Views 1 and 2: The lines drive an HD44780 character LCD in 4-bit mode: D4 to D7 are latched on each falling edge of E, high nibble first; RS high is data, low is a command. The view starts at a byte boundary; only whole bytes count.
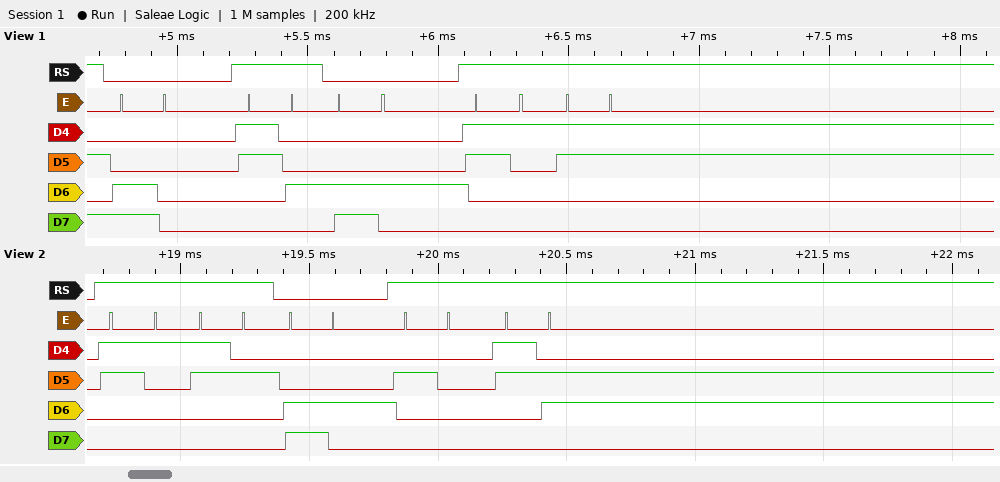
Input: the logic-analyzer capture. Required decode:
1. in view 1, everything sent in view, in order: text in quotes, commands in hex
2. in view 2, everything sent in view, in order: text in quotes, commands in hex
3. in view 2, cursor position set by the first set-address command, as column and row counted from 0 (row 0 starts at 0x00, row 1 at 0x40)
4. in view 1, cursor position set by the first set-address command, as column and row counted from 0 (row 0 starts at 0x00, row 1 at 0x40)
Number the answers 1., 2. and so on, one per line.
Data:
1. 0xC0 "4" 0xC4 "13"
2. "12" 0xC4 " 6"
3. column 4, row 1
4. column 0, row 1
